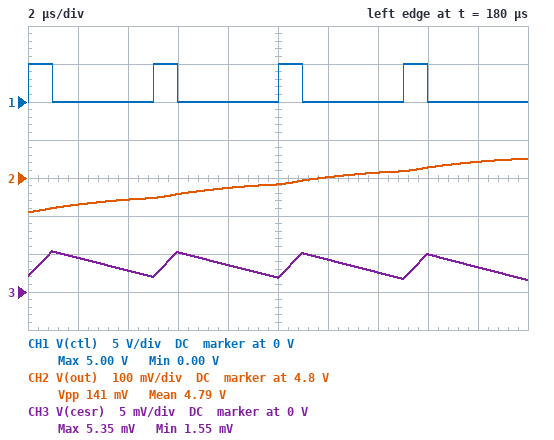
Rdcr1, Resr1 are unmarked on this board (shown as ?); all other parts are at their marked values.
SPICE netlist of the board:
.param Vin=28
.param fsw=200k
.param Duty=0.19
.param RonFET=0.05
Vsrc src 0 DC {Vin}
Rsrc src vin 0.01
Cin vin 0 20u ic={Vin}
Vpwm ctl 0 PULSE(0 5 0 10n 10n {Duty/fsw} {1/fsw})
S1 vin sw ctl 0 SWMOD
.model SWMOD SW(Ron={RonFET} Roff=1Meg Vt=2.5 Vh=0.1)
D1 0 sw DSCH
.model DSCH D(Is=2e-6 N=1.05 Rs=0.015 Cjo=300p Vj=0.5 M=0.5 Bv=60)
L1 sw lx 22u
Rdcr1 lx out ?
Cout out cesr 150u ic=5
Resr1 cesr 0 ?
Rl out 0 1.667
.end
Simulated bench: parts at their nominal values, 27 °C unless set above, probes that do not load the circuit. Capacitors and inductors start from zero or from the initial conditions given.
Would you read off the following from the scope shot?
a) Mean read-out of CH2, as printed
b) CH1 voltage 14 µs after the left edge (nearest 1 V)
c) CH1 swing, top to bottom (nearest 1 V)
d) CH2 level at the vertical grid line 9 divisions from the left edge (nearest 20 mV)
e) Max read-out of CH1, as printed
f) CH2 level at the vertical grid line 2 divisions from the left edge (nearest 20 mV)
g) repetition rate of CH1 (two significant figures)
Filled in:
4.79 V
0 V
5 V
4.84 V
5.00 V
4.74 V
200 kHz
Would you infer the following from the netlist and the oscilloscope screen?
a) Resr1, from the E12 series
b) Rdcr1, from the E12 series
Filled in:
3.3 mΩ
0.068 Ω
